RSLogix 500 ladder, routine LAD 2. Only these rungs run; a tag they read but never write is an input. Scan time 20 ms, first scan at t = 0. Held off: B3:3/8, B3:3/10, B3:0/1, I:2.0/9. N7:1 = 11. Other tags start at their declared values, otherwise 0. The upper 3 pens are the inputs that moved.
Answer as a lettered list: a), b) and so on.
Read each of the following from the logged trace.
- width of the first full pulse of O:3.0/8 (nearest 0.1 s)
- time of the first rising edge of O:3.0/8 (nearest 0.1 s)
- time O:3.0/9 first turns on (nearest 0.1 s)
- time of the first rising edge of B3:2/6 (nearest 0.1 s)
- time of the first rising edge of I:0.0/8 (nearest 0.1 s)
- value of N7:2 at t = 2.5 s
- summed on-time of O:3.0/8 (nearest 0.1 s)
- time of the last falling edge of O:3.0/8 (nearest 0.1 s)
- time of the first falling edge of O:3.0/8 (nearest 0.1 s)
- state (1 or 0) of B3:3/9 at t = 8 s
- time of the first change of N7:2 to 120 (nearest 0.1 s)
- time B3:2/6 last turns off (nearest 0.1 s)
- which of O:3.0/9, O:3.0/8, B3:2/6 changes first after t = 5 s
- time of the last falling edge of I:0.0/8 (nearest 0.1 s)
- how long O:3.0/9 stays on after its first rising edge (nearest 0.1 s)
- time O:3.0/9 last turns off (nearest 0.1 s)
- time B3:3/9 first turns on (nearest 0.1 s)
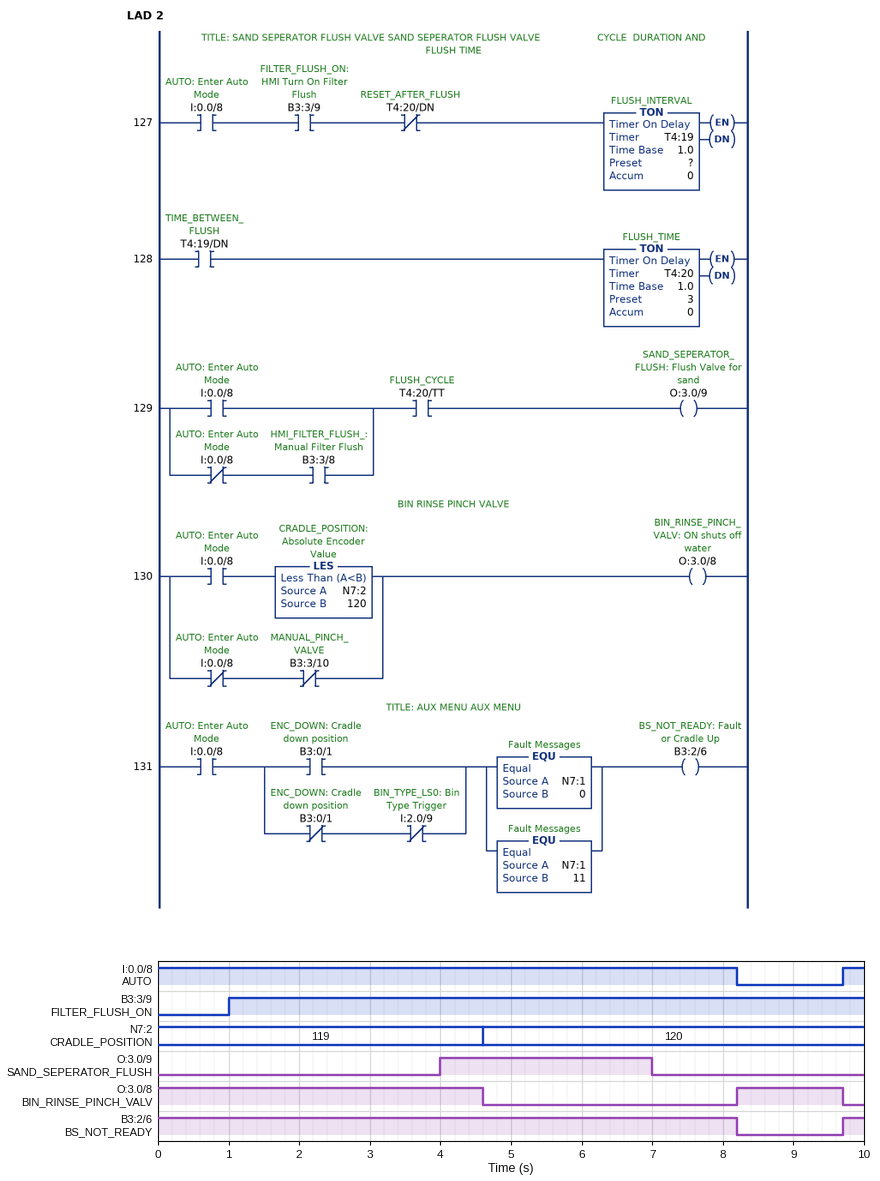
a) 1.5 s
b) 8.2 s
c) 4.0 s
d) 9.7 s
e) 9.7 s
f) 119
g) 6.1 s
h) 9.7 s
i) 4.6 s
j) 1
k) 4.6 s
l) 8.2 s
m) O:3.0/9
n) 8.2 s
o) 3.0 s
p) 7.0 s
q) 1.0 s
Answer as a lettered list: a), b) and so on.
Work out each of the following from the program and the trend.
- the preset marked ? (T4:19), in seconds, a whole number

a) 3 s
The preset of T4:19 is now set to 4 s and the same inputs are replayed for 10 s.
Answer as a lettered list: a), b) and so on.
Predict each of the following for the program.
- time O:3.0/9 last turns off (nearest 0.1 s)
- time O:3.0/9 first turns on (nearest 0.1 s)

a) 8.0 s
b) 5.0 s
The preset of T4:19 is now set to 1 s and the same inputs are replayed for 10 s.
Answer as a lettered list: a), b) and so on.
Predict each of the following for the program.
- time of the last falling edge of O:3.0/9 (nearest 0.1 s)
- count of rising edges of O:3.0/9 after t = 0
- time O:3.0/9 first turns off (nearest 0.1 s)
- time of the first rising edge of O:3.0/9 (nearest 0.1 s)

a) 8.2 s
b) 2
c) 5.0 s
d) 2.0 s
